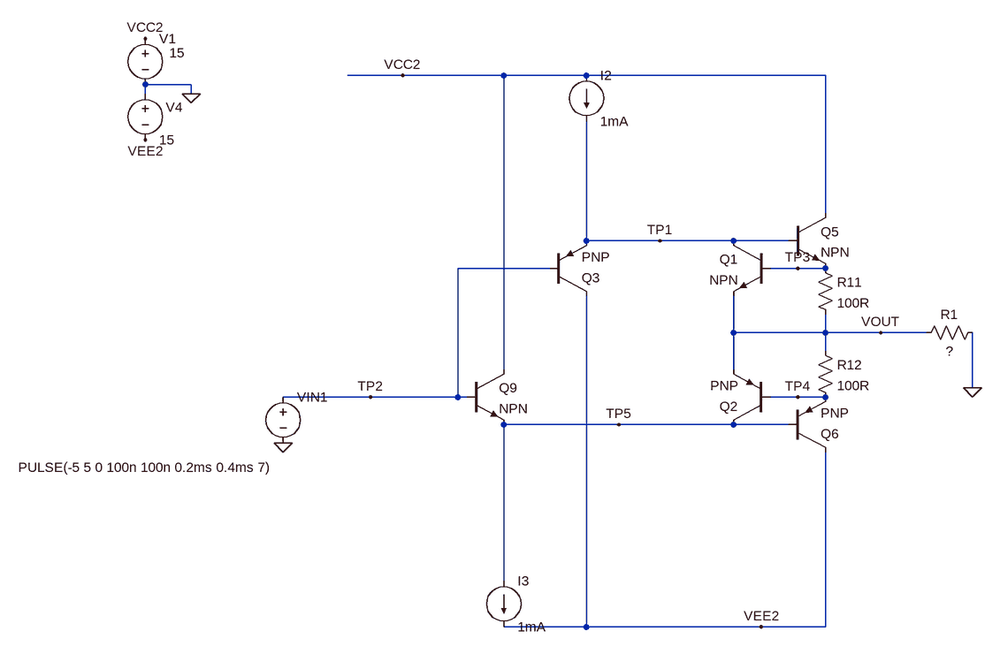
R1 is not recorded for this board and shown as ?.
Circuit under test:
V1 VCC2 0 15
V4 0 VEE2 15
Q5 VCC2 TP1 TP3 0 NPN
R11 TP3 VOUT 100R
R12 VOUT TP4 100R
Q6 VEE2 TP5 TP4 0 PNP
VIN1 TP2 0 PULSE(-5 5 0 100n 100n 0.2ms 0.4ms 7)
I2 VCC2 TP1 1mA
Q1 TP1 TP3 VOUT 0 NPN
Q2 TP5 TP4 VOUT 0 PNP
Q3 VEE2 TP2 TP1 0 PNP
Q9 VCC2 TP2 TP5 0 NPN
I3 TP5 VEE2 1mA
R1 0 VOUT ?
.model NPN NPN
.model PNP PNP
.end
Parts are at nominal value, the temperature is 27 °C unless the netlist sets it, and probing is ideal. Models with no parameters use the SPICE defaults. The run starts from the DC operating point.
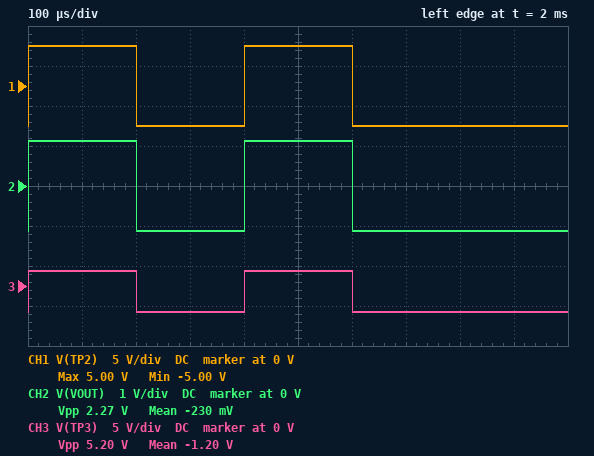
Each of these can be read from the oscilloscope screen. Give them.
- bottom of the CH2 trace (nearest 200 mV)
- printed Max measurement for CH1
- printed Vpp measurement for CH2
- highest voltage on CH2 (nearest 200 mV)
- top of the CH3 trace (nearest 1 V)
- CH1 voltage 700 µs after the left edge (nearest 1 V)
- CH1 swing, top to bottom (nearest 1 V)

-1.2 V
5.00 V
2.27 V
1.2 V
2 V
-5 V
10 V
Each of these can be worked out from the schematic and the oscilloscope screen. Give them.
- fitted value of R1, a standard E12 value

22 Ω
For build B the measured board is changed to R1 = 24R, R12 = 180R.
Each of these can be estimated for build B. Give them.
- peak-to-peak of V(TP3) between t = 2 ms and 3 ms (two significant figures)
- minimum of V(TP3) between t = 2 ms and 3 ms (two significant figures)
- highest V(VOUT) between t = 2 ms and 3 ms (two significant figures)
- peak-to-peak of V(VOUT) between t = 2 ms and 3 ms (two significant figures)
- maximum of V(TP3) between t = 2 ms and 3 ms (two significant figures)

4.9 V
-3.3 V
860 mV
2.0 V
1.6 V
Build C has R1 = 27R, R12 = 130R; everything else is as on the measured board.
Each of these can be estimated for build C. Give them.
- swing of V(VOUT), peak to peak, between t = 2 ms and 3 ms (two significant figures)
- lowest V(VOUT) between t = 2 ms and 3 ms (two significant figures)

2.4 V
-1.3 V
